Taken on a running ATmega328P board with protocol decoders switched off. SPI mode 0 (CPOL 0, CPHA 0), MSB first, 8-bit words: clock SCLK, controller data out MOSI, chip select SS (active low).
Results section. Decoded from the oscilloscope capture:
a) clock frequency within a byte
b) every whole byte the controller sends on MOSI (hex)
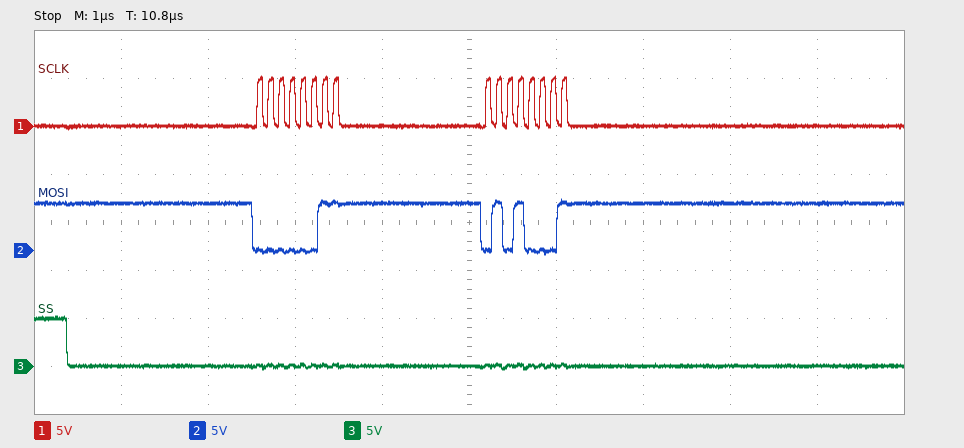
8 MHz
03 51
